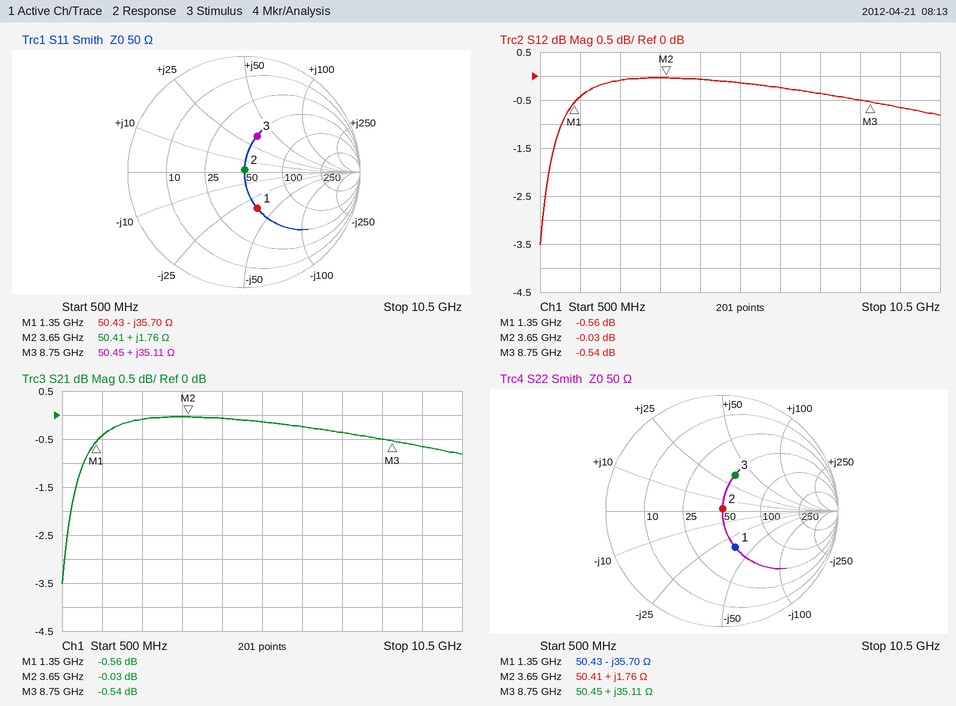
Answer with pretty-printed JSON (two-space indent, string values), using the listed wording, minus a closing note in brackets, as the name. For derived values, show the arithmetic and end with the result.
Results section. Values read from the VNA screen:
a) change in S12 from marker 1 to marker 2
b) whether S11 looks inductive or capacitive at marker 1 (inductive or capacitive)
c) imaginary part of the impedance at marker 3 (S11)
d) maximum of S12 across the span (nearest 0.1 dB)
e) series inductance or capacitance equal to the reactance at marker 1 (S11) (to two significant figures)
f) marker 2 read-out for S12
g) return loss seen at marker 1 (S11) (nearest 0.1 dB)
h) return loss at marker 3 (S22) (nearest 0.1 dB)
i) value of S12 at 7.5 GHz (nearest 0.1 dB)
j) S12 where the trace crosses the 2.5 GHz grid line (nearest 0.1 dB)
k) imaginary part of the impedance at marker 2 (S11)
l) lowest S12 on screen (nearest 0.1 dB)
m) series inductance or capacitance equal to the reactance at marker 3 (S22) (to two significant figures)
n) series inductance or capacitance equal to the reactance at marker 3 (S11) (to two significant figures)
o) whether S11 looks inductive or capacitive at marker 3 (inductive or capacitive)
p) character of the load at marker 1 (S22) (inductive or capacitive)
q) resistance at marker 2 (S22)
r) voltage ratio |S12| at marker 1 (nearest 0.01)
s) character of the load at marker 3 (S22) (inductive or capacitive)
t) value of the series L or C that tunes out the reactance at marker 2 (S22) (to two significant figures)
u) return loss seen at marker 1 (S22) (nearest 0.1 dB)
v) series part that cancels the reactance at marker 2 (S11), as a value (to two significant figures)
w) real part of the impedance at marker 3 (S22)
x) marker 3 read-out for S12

{
  "change in S12 from marker 1 to marker 2": "-0.03 − (-0.56) = 0.53 dB",
  "whether S11 looks inductive or capacitive at marker 1": "capacitive",
  "imaginary part of the impedance at marker 3": "+35.11 Ω",
  "maximum of S12 across the span": "0.0 dB",
  "series inductance or capacitance equal to the reactance at marker 1 (S11)": "C = 1/(2π × 1.35 GHz × 35.7 Ω) ≈ 3.3 pF",
  "marker 2 read-out for S12": "-0.03 dB",
  "return loss seen at marker 1 (S11)": "9.5 dB",
  "return loss at marker 3 (S22)": "9.6 dB",
  "value of S12 at 7.5 GHz": "-0.4 dB",
  "S12 where the trace crosses the 2.5 GHz grid line": "-0.1 dB",
  "imaginary part of the impedance at marker 2": "+1.76 Ω",
  "lowest S12 on screen": "-3.5 dB",
  "series inductance or capacitance equal to the reactance at marker 3 (S22)": "L = 35.11 Ω/(2π × 8.75 GHz) ≈ 639 pH, so 640 pH to two significant figures",
  "series inductance or capacitance equal to the reactance at marker 3 (S11)": "L = 35.11 Ω/(2π × 8.75 GHz) ≈ 639 pH, so 640 pH to two significant figures",
  "whether S11 looks inductive or capacitive at marker 3": "inductive",
  "character of the load at marker 1 (S22)": "capacitive",
  "resistance at marker 2": "50.41 Ω",
  "voltage ratio |S12| at marker 1": "10^(-0.56/20) ≈ 0.94",
  "character of the load at marker 3 (S22)": "inductive",
  "value of the series L or C that tunes out the reactance at marker 2 (S22)": "C = 1/(2π × 3.65 GHz × 1.76 Ω) ≈ 25 pF",
  "return loss seen at marker 1 (S22)": "9.5 dB",
  "series part that cancels the reactance at marker 2 (S11), as a value": "C = 1/(2π × 3.65 GHz × 1.76 Ω) ≈ 25 pF",
  "real part of the impedance at marker 3": "50.45 Ω",
  "marker 3 read-out for S12": "-0.54 dB"
}
